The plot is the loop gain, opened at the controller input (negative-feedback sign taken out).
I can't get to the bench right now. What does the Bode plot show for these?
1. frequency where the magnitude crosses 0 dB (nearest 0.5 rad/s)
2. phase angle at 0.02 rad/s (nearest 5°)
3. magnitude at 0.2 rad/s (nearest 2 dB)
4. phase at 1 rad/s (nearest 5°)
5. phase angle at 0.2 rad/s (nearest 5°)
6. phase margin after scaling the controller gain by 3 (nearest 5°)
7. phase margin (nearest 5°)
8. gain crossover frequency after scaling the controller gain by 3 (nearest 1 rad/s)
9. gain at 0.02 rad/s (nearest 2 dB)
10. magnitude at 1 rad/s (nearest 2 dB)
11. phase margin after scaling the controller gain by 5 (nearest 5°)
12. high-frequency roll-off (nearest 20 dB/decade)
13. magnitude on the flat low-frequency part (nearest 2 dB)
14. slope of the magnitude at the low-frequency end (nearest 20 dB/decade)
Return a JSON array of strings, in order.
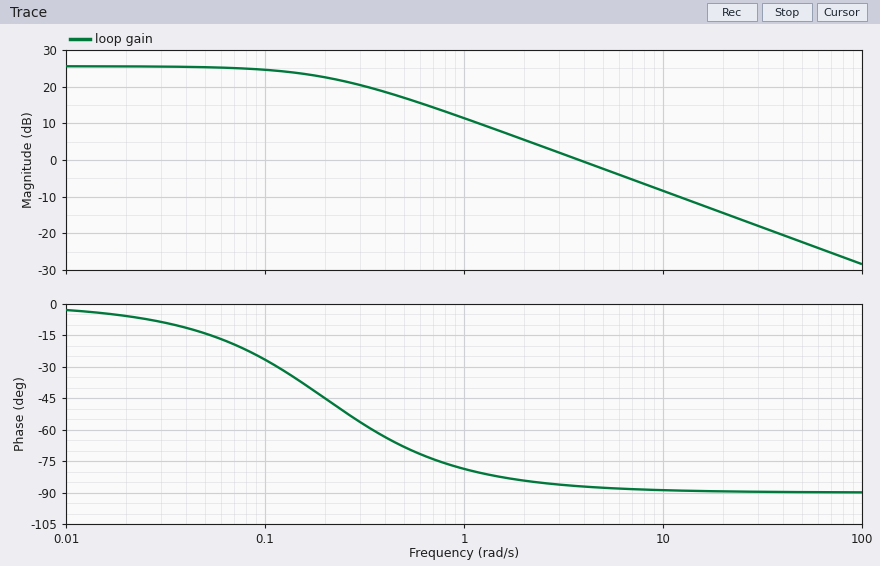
["4.0 rad/s", "-5°", "22 dB", "-80°", "-45°", "90°", "95°", "11 rad/s", "26 dB", "12 dB", "90°", "-20 dB/decade", "26 dB", "0 dB/decade"]
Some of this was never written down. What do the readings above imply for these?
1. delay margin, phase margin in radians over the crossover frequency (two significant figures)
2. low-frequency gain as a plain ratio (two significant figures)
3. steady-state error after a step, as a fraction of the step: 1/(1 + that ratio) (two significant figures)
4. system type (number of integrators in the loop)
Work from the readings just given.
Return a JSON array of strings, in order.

["0.41 s", "20", "0.048", "0"]
